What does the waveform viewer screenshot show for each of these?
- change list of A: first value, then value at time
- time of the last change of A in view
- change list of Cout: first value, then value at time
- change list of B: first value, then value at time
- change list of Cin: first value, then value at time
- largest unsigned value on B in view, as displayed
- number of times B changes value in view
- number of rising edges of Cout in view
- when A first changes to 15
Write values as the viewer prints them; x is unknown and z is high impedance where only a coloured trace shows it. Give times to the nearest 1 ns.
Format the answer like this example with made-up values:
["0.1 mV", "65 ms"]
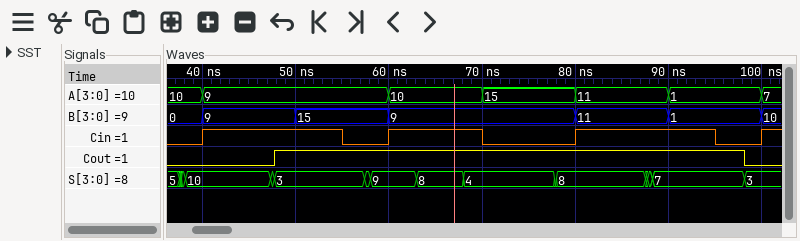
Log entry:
["10, 9 at 40 ns, 10 at 60 ns, 15 at 70 ns, 11 at 80 ns, 1 at 90 ns, 7 at 100 ns", "100 ns", "0, 1 at 48 ns, 0 at 98 ns", "0, 9 at 40 ns, 15 at 50 ns, 9 at 60 ns, 11 at 80 ns, 1 at 90 ns, 10 at 100 ns", "0, 1 at 40 ns, 0 at 55 ns, 1 at 60 ns, 0 at 70 ns, 1 at 80 ns, 0 at 95 ns, 1 at 100 ns", "15", "6", "1", "70 ns"]
